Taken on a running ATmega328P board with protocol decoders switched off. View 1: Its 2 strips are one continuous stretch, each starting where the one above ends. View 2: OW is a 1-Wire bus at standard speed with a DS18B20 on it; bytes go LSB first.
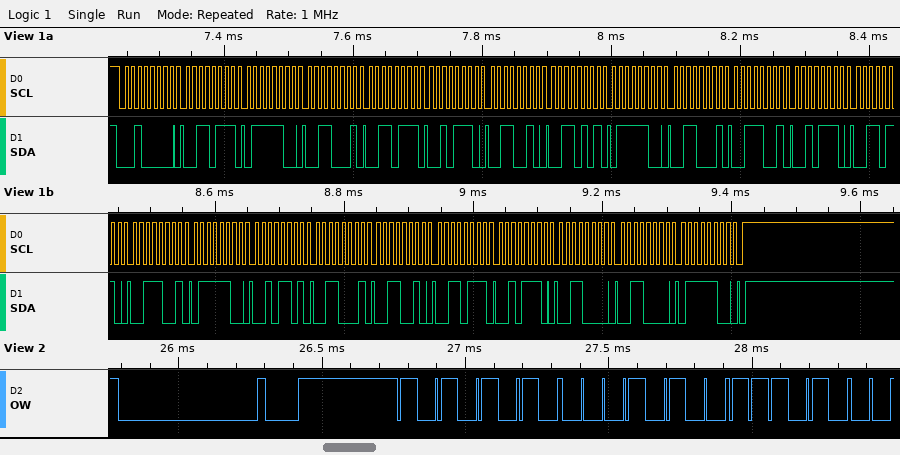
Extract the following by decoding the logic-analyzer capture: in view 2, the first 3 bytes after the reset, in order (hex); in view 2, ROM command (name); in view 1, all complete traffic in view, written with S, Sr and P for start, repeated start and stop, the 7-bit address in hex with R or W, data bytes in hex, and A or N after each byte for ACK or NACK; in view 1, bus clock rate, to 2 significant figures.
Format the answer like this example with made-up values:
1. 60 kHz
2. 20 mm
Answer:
1. 55 28 17
2. Match ROM
3. S 10W A 37 A 7C A 31 A 37 A 2E A 32 A 35 A 7C A 31 A 39 A 2E A 36 A 39 A 7C A 2D A 31 A 32 A 37 A 2E A 30 A 30 A 7C A P
4. 100 kHz
